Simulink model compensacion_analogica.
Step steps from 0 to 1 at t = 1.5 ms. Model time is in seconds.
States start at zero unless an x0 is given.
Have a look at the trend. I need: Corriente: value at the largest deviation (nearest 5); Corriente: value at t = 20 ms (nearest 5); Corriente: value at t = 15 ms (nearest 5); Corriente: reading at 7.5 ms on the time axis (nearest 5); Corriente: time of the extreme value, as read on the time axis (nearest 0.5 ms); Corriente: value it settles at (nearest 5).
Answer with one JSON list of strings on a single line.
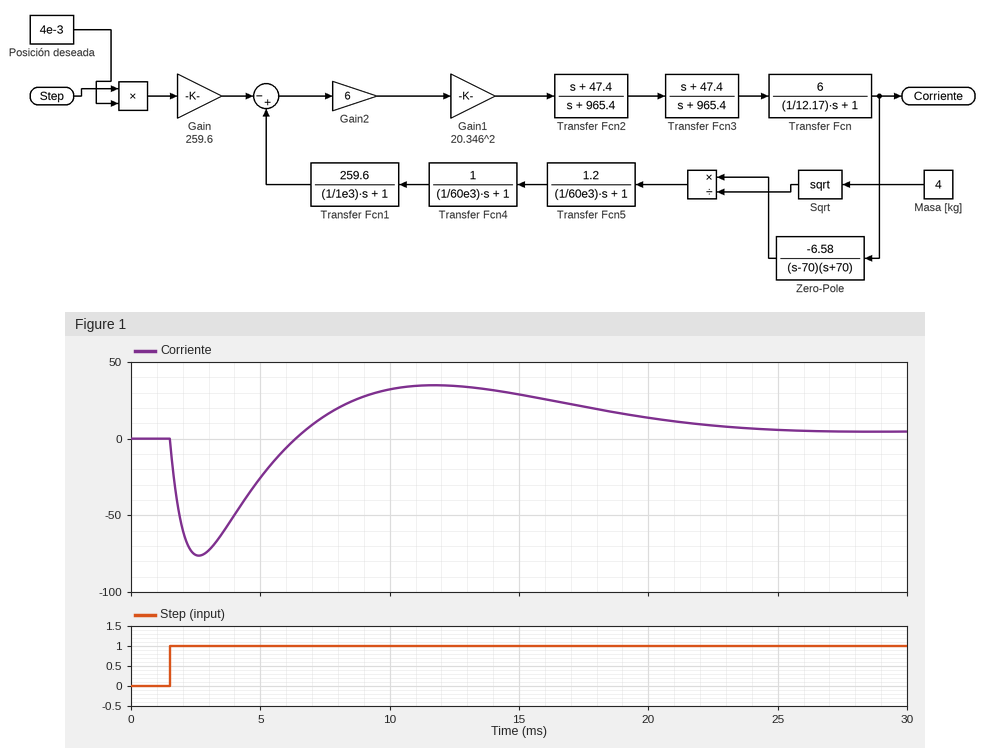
["-75", "15", "30", "15", "2.5 ms", "5"]
